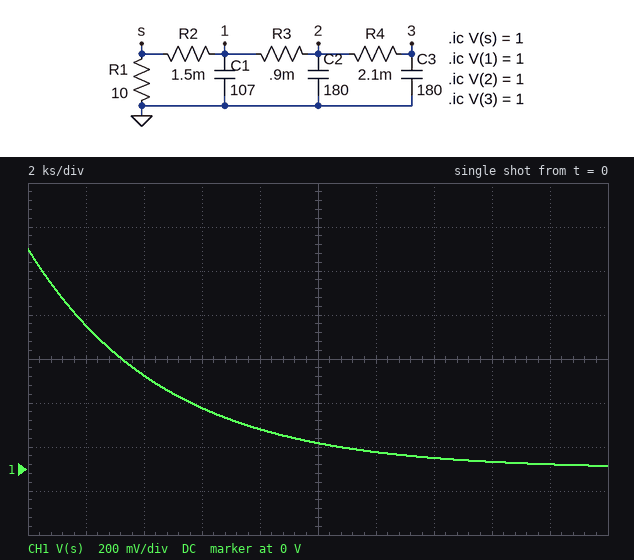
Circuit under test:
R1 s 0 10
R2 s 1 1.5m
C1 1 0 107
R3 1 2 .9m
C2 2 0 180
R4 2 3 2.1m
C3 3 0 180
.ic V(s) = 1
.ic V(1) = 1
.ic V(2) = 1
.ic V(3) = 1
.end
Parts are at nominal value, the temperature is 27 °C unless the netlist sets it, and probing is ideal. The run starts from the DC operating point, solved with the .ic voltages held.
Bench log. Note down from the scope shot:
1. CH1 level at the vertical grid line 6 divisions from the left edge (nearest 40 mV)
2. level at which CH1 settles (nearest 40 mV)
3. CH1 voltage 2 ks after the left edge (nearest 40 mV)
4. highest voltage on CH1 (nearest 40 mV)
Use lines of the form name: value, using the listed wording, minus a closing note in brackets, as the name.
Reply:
CH1 level at the vertical grid line 6 divisions from the left edge: 80 mV
level at which CH1 settles: 0 V
CH1 voltage 2 ks after the left edge: 640 mV
highest voltage on CH1: 1.00 V
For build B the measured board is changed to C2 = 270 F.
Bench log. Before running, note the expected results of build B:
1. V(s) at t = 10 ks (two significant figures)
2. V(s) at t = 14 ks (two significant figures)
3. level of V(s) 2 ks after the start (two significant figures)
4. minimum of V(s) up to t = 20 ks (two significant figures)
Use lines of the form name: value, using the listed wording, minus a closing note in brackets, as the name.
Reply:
V(s) at t = 10 ks: 170 mV
V(s) at t = 14 ks: 81 mV
level of V(s) 2 ks after the start: 700 mV
minimum of V(s) up to t = 20 ks: 28 mV
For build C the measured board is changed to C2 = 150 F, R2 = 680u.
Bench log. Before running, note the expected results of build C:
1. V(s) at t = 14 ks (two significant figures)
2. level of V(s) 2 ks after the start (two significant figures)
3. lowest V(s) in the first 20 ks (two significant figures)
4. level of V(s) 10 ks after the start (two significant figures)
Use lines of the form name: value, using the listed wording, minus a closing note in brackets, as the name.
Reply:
V(s) at t = 14 ks: 41 mV
level of V(s) 2 ks after the start: 630 mV
lowest V(s) in the first 20 ks: 10 mV
level of V(s) 10 ks after the start: 100 mV
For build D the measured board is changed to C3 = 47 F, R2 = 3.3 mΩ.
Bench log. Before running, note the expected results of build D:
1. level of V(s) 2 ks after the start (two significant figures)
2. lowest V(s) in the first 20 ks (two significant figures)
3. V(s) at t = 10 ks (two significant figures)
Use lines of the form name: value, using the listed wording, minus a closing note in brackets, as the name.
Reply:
level of V(s) 2 ks after the start: 550 mV
lowest V(s) in the first 20 ks: 2.5 mV
V(s) at t = 10 ks: 50 mV
